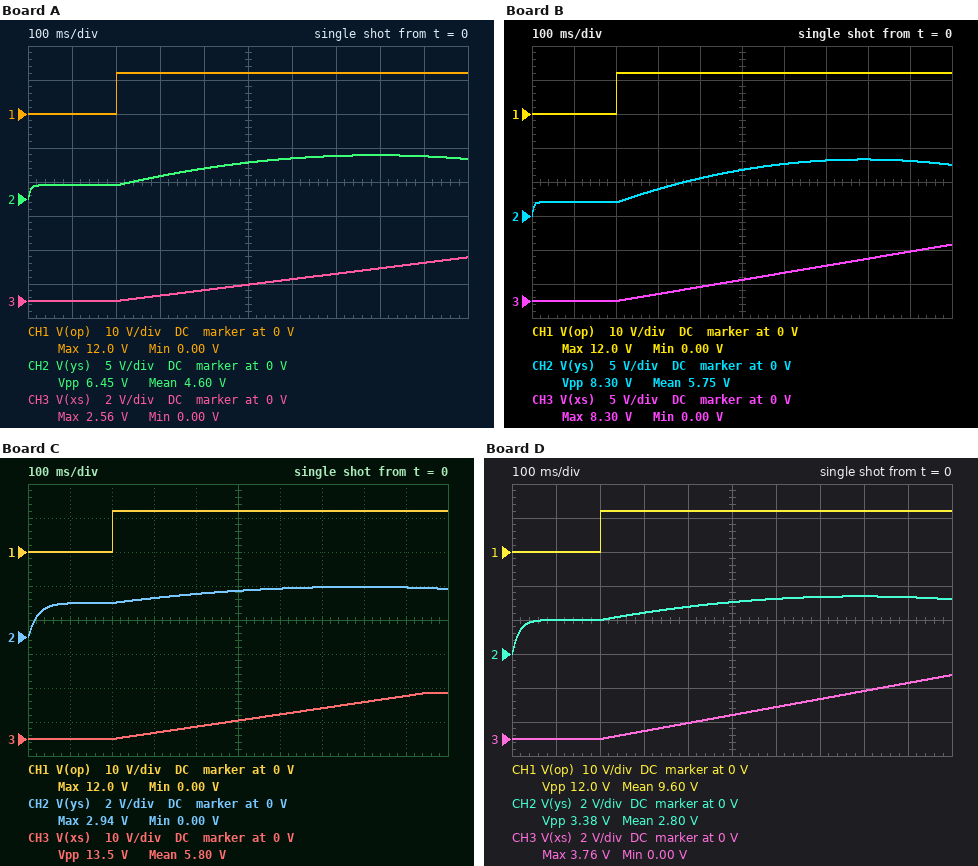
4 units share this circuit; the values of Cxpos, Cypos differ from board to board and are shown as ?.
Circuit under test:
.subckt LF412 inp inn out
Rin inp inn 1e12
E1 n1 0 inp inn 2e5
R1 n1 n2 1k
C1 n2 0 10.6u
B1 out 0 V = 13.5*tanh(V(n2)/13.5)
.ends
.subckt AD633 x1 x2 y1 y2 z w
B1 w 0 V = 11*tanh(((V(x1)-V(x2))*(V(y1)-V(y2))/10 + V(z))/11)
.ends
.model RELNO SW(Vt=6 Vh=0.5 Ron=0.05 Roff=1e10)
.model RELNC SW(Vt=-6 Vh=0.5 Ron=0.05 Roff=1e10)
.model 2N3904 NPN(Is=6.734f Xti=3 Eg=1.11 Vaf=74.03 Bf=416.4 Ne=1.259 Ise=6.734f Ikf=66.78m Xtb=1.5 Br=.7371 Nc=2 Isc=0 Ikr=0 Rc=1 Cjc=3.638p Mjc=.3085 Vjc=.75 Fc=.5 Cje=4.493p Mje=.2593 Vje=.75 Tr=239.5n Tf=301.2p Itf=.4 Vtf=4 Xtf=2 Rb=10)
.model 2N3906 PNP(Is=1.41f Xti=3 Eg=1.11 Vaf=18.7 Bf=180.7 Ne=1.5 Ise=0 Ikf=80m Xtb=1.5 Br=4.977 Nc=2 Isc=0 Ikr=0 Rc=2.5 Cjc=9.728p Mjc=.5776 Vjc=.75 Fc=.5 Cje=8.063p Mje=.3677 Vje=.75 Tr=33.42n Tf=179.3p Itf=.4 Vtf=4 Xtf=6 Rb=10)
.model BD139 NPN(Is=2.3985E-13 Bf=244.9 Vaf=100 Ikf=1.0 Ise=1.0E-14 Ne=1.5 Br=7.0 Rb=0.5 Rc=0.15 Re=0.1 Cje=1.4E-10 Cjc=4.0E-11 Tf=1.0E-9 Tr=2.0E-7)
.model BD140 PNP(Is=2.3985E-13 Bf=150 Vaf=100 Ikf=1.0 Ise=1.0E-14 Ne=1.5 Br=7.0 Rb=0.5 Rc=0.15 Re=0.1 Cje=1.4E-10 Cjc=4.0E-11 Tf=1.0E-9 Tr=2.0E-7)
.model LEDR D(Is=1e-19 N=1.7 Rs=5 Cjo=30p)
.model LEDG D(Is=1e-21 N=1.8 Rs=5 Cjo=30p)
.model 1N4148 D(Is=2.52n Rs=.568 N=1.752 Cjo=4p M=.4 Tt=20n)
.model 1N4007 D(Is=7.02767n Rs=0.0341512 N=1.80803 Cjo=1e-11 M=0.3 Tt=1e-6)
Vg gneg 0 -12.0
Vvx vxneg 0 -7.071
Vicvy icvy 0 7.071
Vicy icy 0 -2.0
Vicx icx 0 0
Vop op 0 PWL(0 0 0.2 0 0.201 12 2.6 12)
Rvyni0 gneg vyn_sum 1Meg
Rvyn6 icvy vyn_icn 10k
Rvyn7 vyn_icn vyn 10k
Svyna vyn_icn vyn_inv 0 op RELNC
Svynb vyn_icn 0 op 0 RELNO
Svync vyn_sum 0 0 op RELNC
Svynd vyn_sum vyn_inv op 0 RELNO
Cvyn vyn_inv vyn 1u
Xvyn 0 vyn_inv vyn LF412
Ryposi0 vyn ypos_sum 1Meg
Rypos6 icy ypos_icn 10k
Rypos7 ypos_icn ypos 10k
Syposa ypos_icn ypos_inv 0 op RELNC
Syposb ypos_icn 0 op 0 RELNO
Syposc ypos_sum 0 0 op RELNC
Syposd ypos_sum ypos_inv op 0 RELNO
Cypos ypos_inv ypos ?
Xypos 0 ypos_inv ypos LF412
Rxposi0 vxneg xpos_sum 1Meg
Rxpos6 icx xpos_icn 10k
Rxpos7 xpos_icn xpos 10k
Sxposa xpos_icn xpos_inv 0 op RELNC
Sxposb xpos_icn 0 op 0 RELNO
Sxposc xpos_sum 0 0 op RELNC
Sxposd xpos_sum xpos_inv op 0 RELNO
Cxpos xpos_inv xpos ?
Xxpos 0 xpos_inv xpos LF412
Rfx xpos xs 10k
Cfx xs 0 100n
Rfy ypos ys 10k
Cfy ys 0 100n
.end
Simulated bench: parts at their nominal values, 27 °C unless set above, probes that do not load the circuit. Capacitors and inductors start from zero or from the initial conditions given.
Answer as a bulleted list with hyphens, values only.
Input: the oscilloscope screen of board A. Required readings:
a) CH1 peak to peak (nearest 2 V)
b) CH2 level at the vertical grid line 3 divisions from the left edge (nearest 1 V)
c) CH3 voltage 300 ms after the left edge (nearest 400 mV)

- 12 V
- 3 V
- 400 mV
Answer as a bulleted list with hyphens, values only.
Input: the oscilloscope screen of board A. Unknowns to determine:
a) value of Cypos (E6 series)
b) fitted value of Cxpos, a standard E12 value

- 470 nF
- 2.2 µF
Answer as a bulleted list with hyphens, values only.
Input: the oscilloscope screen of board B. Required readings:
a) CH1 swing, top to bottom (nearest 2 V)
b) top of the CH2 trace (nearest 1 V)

- 12 V
- 8 V
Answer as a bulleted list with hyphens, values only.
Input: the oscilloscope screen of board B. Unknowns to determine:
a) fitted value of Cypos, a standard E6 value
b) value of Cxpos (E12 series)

- 330 nF
- 680 nF
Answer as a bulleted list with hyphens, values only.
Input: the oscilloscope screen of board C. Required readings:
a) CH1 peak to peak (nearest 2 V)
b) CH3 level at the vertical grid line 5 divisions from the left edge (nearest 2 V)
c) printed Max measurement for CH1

- 12 V
- 6 V
- 12.0 V
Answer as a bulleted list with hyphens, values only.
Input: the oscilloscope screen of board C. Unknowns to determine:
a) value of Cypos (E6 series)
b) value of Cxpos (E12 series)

- 2.2 µF
- 390 nF
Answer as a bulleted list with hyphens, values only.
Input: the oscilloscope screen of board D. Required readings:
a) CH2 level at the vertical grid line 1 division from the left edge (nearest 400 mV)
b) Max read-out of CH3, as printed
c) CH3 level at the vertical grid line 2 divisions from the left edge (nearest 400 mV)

- 2.0 V
- 3.76 V
- 0 V
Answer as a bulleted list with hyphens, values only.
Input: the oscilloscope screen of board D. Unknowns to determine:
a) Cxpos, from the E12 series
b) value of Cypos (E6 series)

- 1.5 µF
- 1.5 µF
